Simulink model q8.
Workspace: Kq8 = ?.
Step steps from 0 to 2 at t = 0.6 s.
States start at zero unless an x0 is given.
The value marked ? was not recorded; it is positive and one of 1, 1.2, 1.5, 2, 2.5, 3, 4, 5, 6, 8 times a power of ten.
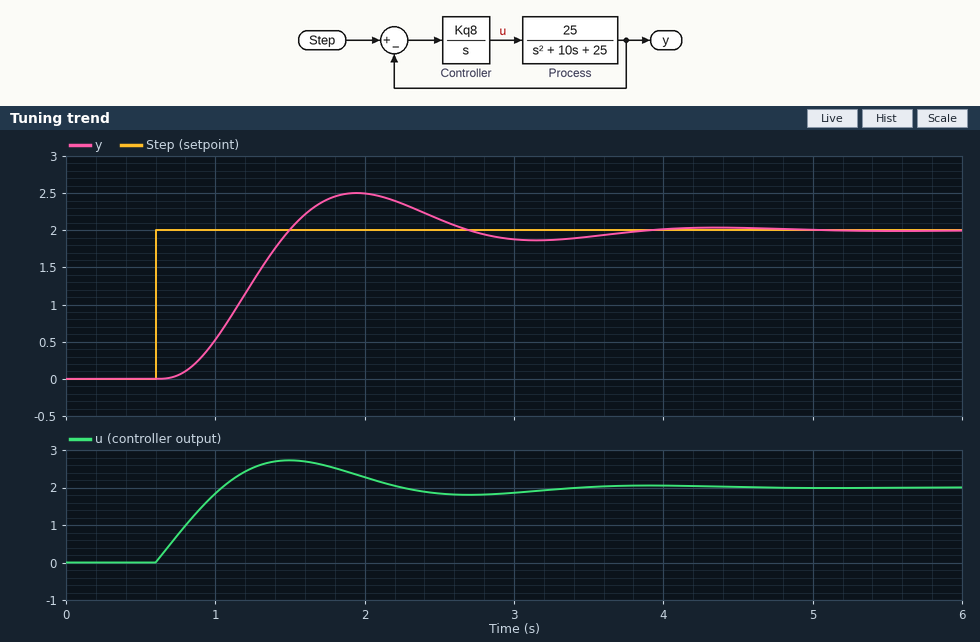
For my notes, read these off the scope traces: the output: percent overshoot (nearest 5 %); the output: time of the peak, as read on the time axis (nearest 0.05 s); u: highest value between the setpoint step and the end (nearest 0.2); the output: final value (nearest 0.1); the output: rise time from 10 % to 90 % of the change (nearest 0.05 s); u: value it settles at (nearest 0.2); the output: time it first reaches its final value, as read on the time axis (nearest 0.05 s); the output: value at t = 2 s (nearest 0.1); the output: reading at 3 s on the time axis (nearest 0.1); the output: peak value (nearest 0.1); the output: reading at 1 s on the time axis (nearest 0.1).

25 %
1.95 s
2.8
2.0
0.55 s
2.0
1.50 s
2.5
1.9
2.5
0.5
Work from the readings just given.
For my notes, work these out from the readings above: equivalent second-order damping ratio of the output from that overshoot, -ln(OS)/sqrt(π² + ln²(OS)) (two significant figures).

0.40
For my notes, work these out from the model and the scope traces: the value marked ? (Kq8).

2.5
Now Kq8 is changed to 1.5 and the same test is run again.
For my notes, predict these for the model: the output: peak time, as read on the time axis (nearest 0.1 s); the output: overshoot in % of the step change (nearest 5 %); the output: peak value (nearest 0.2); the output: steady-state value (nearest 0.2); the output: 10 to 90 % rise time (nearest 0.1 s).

2.5 s
10 %
2.2
2.0
0.9 s
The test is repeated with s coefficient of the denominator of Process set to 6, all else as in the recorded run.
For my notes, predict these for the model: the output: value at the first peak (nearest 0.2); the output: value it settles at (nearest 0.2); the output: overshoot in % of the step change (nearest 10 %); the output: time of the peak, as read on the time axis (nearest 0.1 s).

2.4
2.0
20 %
1.7 s
